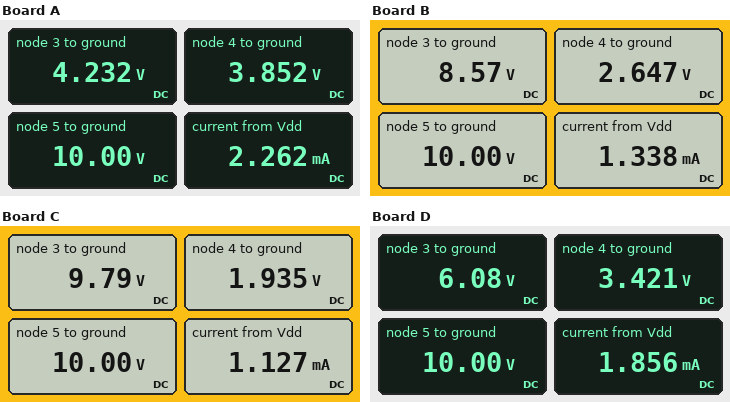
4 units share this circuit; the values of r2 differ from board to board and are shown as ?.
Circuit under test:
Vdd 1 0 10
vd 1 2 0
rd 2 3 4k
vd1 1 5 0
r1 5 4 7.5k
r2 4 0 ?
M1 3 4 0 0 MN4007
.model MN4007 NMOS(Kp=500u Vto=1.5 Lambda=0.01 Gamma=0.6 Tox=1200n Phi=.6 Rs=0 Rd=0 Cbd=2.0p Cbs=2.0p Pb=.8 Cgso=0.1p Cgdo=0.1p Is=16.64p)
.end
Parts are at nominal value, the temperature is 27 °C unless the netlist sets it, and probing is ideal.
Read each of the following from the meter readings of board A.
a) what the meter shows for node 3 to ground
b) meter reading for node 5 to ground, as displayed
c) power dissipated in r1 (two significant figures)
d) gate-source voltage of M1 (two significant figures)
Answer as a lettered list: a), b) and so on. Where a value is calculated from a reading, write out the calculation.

a) 4.232 V
b) 10.00 V
c) (10 V - 3.852 V)^2 / 7.5 kΩ = 5.0 mW
d) 3.852 V = 3.9 V
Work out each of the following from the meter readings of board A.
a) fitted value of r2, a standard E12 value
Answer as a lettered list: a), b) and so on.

a) 4.7 kΩ
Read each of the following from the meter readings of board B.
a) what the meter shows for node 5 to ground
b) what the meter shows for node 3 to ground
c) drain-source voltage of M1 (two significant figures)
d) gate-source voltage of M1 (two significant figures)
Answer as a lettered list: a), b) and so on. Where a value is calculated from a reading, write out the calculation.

a) 10.00 V
b) 8.57 V
c) 8.57 V = 8.6 V
d) 2.647 V = 2.6 V
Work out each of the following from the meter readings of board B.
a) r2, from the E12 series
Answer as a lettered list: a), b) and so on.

a) 2.7 kΩ
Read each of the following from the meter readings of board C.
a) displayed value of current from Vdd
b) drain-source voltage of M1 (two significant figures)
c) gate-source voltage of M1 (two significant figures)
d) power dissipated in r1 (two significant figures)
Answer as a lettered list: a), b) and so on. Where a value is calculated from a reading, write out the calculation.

a) 1.127 mA
b) 9.79 V = 9.8 V
c) 1.935 V = 1.9 V
d) (10 V - 1.935 V)^2 / 7.5 kΩ = 8.7 mW
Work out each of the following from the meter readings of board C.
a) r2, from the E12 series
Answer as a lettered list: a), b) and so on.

a) 1.8 kΩ
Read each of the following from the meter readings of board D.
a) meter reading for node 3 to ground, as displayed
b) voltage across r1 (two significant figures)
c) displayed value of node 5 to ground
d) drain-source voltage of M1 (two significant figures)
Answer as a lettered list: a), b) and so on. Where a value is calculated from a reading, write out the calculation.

a) 6.08 V
b) 10 V - 3.421 V = 6.6 V
c) 10.00 V
d) 6.08 V = 6.1 V
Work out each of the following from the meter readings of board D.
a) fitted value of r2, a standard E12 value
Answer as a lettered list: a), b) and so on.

a) 3.9 kΩ
